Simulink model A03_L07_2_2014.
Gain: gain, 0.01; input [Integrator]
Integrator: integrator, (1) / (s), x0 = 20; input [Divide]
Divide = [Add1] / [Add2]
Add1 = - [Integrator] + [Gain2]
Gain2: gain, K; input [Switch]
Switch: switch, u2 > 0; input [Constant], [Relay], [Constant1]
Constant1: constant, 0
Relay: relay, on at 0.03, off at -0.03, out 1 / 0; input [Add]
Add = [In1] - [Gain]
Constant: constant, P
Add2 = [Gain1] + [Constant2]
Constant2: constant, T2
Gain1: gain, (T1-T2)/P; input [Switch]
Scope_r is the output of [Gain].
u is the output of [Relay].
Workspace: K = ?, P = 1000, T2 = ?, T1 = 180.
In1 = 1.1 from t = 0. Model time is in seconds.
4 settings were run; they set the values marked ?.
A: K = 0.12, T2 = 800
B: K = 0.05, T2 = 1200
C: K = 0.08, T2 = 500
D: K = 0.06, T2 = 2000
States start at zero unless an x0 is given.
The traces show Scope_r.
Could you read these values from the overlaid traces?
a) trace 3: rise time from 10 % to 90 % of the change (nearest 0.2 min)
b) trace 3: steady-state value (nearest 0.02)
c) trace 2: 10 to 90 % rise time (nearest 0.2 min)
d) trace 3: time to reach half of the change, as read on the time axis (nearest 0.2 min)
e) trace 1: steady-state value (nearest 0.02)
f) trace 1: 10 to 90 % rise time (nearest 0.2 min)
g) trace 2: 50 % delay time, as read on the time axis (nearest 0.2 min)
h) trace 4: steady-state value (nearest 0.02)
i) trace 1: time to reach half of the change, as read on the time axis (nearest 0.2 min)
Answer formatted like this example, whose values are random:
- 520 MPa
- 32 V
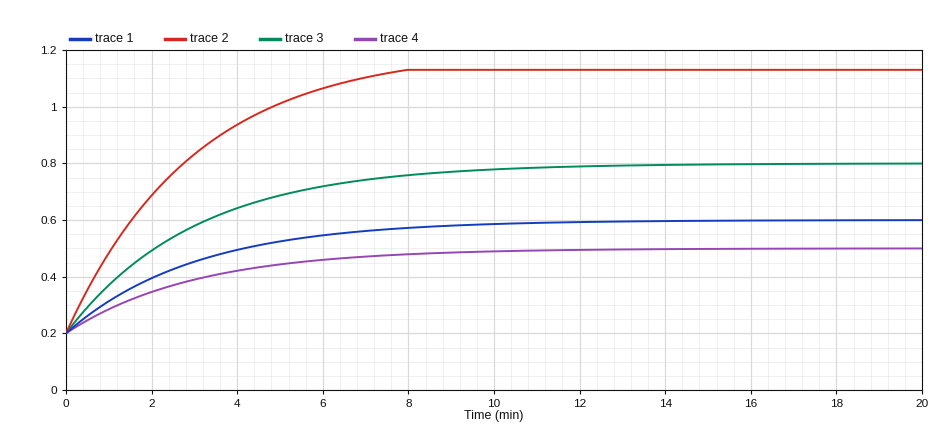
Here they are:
- 6.6 min
- 0.80
- 5.2 min
- 2.0 min
- 0.60
- 6.6 min
- 1.8 min
- 0.50
- 2.0 min
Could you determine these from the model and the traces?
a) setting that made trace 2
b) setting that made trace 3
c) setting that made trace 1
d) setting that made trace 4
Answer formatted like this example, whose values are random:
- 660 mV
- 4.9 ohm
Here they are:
- A
- C
- D
- B
